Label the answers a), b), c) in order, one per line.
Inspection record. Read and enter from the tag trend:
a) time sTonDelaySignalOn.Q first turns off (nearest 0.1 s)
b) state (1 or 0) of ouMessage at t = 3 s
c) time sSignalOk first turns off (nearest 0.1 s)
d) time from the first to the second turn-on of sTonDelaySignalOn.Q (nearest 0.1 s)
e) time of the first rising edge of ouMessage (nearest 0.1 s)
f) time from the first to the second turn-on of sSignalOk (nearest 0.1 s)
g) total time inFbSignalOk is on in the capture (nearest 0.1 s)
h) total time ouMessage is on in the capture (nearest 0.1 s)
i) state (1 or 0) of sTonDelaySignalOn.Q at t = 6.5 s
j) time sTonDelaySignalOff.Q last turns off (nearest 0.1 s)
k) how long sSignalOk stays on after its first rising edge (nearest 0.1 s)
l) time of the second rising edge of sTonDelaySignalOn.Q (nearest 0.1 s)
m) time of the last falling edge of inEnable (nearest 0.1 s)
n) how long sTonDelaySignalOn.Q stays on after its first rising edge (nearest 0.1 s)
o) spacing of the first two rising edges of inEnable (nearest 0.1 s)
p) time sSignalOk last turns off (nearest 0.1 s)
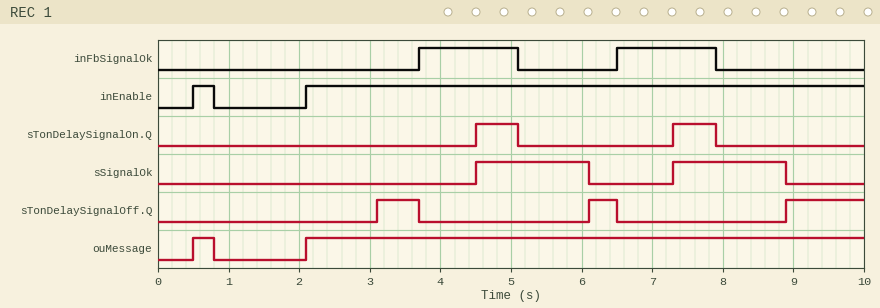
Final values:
a) 5.1 s
b) 1
c) 6.1 s
d) 2.8 s
e) 0.5 s
f) 2.8 s
g) 2.8 s
h) 8.2 s
i) 0
j) 6.5 s
k) 1.6 s
l) 7.3 s
m) 0.8 s
n) 0.6 s
o) 1.6 s
p) 8.9 s
